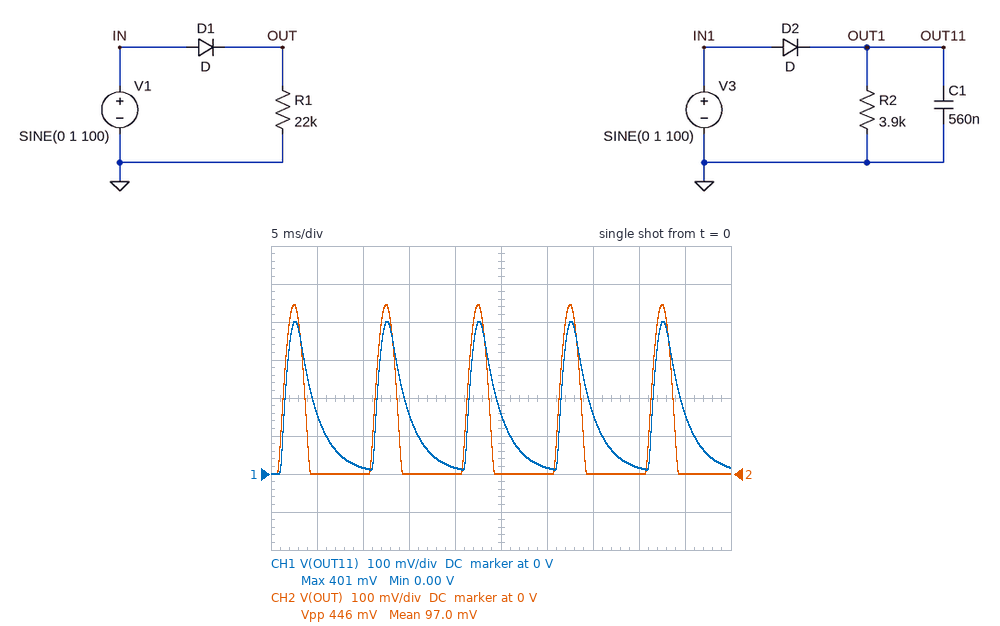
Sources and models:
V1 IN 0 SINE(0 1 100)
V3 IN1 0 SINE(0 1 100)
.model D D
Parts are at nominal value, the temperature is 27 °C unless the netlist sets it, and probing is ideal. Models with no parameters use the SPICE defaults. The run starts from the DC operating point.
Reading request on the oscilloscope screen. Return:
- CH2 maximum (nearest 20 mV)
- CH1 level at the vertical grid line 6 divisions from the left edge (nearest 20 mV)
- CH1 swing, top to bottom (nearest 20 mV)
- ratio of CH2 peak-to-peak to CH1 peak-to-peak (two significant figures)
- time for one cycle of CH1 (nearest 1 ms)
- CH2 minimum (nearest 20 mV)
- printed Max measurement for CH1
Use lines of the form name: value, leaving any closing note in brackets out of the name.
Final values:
CH2 maximum: 440 mV
CH1 level at the vertical grid line 6 divisions from the left edge: 20 mV
CH1 swing, top to bottom: 400 mV
ratio of CH2 peak-to-peak to CH1 peak-to-peak: 1.1
time for one cycle of CH1: 10 ms
CH2 minimum: 0 V
printed Max measurement for CH1: 401 mV
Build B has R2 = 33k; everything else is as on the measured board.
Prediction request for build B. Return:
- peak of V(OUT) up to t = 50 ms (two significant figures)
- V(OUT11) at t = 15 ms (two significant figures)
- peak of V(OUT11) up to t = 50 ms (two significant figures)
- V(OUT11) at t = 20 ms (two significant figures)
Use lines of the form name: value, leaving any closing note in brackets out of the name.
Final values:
peak of V(OUT) up to t = 50 ms: 450 mV
V(OUT11) at t = 15 ms: 390 mV
peak of V(OUT11) up to t = 50 ms: 430 mV
V(OUT11) at t = 20 ms: 300 mV
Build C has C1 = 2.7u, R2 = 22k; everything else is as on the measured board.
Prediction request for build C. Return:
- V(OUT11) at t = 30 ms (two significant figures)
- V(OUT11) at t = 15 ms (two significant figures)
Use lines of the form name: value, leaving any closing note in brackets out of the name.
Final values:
V(OUT11) at t = 30 ms: 360 mV
V(OUT11) at t = 15 ms: 390 mV
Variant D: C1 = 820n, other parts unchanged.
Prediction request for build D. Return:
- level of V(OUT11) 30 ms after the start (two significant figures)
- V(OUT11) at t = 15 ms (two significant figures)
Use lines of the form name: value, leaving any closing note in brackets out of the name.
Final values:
level of V(OUT11) 30 ms after the start: 44 mV
V(OUT11) at t = 15 ms: 210 mV
